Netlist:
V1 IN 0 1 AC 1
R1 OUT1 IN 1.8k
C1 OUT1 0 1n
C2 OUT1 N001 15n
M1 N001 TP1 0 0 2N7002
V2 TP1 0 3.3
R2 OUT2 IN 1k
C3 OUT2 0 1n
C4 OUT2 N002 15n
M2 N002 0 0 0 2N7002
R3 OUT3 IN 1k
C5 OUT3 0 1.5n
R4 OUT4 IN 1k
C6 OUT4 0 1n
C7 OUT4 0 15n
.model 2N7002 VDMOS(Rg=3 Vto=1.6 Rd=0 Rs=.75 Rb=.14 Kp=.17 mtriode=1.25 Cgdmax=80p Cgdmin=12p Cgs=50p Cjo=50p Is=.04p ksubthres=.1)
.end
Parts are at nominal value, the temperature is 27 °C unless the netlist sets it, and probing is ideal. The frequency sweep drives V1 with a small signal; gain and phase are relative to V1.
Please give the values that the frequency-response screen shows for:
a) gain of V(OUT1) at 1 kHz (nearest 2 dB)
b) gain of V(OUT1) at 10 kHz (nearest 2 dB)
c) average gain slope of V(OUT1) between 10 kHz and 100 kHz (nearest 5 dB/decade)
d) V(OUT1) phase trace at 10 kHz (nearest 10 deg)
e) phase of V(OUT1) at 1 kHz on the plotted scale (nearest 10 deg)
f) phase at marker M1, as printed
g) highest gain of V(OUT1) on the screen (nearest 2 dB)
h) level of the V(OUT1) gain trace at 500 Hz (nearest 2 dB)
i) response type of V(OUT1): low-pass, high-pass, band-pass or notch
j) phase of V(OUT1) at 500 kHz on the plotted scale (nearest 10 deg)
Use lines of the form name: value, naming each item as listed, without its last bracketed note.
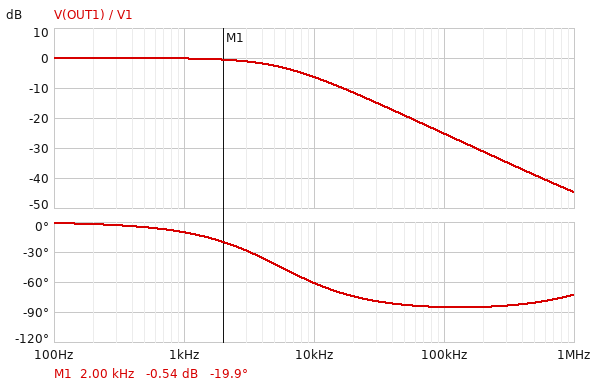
gain of V(OUT1) at 1 kHz: 0 dB
gain of V(OUT1) at 10 kHz: -6 dB
average gain slope of V(OUT1) between 10 kHz and 100 kHz: -20 dB/decade
V(OUT1) phase trace at 10 kHz: -60 deg
phase of V(OUT1) at 1 kHz on the plotted scale: -10 deg
phase at marker M1, as printed: -19.9 deg
highest gain of V(OUT1) on the screen: 0 dB
level of the V(OUT1) gain trace at 500 Hz: 0 dB
response type of V(OUT1): low-pass, high-pass, band-pass or notch: low-pass
phase of V(OUT1) at 500 kHz on the plotted scale: -80 deg
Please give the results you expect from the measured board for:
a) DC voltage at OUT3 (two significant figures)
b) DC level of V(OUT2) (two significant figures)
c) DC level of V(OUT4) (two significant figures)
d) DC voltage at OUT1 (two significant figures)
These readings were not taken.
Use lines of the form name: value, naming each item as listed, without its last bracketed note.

DC voltage at OUT3: 1.0 V
DC level of V(OUT2): 1.0 V
DC level of V(OUT4): 1.0 V
DC voltage at OUT1: 1.0 V
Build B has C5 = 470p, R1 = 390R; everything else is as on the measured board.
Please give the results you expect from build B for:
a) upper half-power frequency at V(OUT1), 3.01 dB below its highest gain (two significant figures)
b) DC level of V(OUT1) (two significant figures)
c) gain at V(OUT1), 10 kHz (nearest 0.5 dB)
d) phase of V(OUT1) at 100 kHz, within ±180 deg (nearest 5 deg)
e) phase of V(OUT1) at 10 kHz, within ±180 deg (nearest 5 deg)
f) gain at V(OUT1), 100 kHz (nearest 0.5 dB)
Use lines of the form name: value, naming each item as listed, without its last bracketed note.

upper half-power frequency at V(OUT1), 3.01 dB below its highest gain: 25 kHz
DC level of V(OUT1): 1.0 V
gain at V(OUT1), 10 kHz: -0.5 dB
phase of V(OUT1) at 100 kHz, within ±180 deg: -75 deg
phase of V(OUT1) at 10 kHz, within ±180 deg: -20 deg
gain at V(OUT1), 100 kHz: -12.0 dB
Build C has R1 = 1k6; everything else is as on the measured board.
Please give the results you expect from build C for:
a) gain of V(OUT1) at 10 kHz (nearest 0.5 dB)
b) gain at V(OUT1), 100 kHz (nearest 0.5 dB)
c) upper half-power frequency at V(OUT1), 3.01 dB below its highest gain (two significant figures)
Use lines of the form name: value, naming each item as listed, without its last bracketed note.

gain of V(OUT1) at 10 kHz: -5.5 dB
gain at V(OUT1), 100 kHz: -24.0 dB
upper half-power frequency at V(OUT1), 3.01 dB below its highest gain: 6.2 kHz
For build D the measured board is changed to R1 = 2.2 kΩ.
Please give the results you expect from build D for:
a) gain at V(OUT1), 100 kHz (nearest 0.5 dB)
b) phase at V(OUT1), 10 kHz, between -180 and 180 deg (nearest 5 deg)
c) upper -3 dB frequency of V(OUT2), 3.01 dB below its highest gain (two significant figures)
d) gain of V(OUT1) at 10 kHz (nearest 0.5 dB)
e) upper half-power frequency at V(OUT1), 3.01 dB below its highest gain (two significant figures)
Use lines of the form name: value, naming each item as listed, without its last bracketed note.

gain at V(OUT1), 100 kHz: -27.0 dB
phase at V(OUT1), 10 kHz, between -180 and 180 deg: -65 deg
upper -3 dB frequency of V(OUT2), 3.01 dB below its highest gain: 140 kHz
gain of V(OUT1) at 10 kHz: -7.5 dB
upper half-power frequency at V(OUT1), 3.01 dB below its highest gain: 4.5 kHz
